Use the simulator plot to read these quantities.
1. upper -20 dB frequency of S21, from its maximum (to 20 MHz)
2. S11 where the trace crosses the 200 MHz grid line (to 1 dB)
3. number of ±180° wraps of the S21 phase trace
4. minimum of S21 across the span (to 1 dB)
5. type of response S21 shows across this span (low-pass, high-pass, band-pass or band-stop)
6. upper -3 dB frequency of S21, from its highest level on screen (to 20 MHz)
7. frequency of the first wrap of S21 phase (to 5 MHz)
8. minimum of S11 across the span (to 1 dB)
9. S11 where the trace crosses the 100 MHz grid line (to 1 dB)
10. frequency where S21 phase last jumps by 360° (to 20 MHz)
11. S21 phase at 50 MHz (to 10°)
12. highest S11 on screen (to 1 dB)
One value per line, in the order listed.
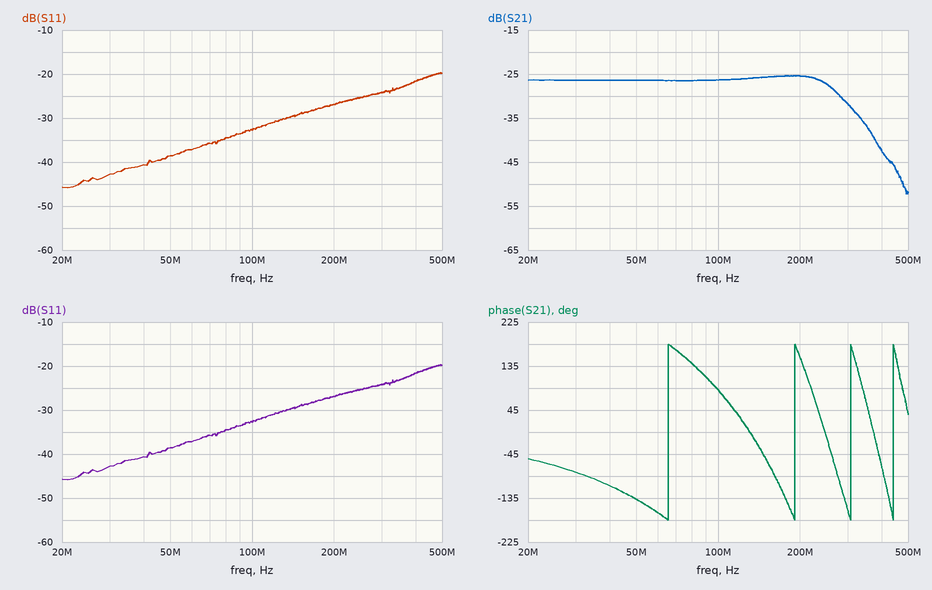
440 MHz
-27 dB
4
-52 dB
low-pass
260 MHz
65 MHz
-46 dB
-33 dB
440 MHz
-140°
-20 dB
